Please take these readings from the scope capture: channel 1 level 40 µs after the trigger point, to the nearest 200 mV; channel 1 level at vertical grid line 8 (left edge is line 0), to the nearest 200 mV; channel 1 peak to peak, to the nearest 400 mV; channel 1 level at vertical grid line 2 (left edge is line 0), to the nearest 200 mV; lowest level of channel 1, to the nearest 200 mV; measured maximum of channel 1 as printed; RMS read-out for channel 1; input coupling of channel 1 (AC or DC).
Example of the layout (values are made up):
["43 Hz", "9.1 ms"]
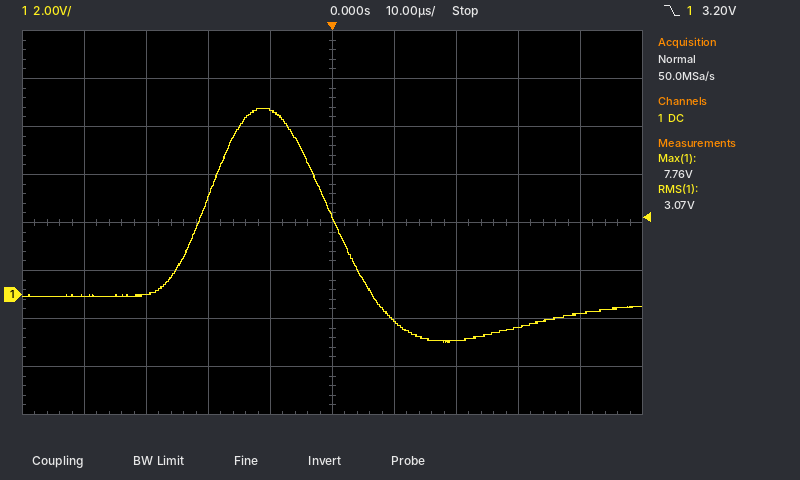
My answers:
["-800 mV", "-1.4 V", "9.6 V", "0.0 V", "-2.0 V", "7.76 V", "3.07 V", "DC"]
